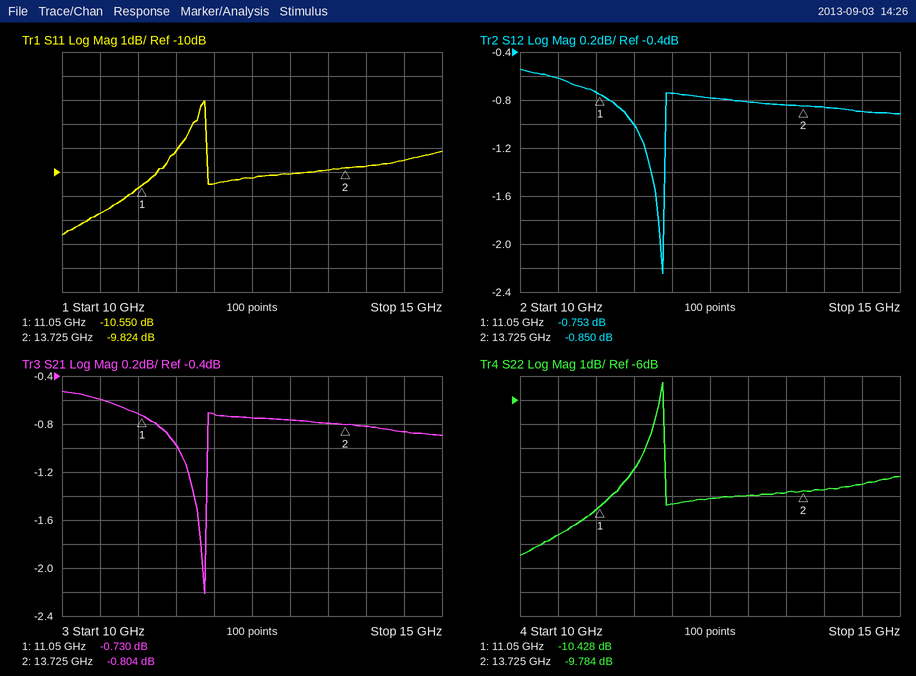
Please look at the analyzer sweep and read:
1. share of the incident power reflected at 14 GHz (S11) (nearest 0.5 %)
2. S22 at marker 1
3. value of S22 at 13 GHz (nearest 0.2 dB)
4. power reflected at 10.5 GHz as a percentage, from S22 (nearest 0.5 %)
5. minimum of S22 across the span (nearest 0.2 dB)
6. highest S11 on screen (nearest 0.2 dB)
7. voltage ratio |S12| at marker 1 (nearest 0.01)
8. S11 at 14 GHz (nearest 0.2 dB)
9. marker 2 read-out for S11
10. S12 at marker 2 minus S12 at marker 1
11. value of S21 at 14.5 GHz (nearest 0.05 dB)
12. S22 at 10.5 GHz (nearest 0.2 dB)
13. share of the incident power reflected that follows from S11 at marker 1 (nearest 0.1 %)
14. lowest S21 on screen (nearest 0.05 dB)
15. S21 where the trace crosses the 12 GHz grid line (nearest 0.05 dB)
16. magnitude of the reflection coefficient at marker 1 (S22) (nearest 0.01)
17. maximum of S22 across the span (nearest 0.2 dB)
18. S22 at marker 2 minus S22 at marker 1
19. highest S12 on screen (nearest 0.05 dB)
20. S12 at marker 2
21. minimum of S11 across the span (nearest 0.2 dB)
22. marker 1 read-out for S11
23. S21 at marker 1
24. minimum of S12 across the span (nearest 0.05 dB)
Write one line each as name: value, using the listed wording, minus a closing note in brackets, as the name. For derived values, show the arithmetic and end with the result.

share of the incident power reflected at 14 GHz (S11): 10^(-9.8/10) ≈ 10.5 %
S22 at marker 1: -10.428 dB
value of S22 at 13 GHz: -10.0 dB
power reflected at 10.5 GHz as a percentage, from S22: 10^(-11.6/10) ≈ 6.92 %, so 7.0 % to the nearest 0.5 %
minimum of S22 across the span: -12.4 dB
highest S11 on screen: -7.0 dB
voltage ratio |S12| at marker 1: 10^(-0.753/20) ≈ 0.92
S11 at 14 GHz: -9.8 dB
marker 2 read-out for S11: -9.824 dB
S12 at marker 2 minus S12 at marker 1: -0.85 − (-0.753) = -0.097 dB
value of S21 at 14.5 GHz: -0.85 dB
S22 at 10.5 GHz: -11.6 dB
share of the incident power reflected that follows from S11 at marker 1: 10^(-10.55/10) ≈ 8.8 %
lowest S21 on screen: -2.20 dB
S21 where the trace crosses the 12 GHz grid line: -0.70 dB
magnitude of the reflection coefficient at marker 1 (S22): 10^(-10.428/20) ≈ 0.30
maximum of S22 across the span: -5.2 dB
S22 at marker 2 minus S22 at marker 1: -9.784 − (-10.428) = 0.644 dB
highest S12 on screen: -0.55 dB
S12 at marker 2: -0.850 dB
minimum of S11 across the span: -12.6 dB
marker 1 read-out for S11: -10.550 dB
S21 at marker 1: -0.730 dB
minimum of S12 across the span: -2.25 dB
